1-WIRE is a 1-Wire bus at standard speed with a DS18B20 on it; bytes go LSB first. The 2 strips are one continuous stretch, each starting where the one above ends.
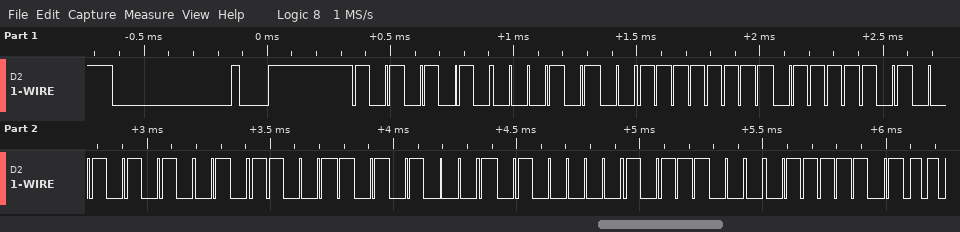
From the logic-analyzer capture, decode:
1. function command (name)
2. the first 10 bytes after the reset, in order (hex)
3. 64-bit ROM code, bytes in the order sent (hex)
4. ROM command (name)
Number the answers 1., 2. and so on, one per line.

1. Read Scratchpad
2. 55 28 FF BE 54 9A 15 05 1D BE
3. 28 FF BE 54 9A 15 05 1D
4. Match ROM
